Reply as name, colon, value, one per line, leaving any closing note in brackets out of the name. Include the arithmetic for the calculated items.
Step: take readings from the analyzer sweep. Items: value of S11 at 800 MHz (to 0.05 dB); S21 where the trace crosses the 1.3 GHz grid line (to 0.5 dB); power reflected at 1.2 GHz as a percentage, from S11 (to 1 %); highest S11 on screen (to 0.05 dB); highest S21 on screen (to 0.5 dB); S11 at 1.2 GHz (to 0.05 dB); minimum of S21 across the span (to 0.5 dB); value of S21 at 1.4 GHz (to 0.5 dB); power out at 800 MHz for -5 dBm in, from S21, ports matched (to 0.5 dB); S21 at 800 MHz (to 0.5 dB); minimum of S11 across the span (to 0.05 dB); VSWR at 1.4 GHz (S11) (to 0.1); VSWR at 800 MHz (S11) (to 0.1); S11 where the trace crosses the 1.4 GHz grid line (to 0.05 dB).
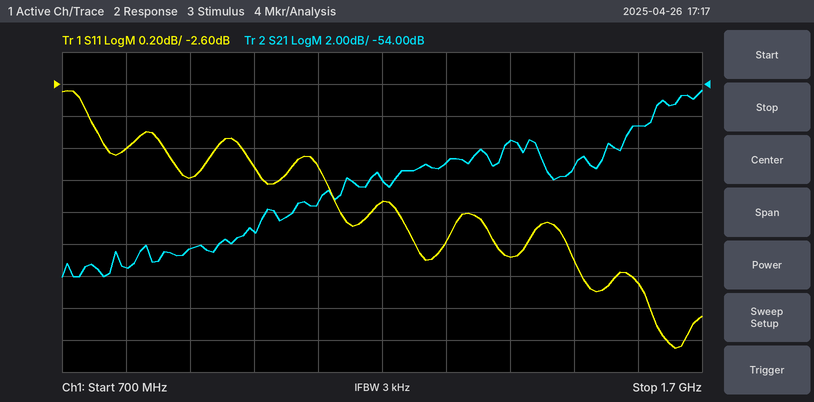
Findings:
value of S11 at 800 MHz: -3.00 dB
S21 where the trace crosses the 1.3 GHz grid line: -59.0 dB
power reflected at 1.2 GHz as a percentage, from S11: 10^(-3.35/10) ≈ 46 %
highest S11 on screen: -2.65 dB
highest S21 on screen: -54.5 dB
S11 at 1.2 GHz: -3.35 dB
minimum of S21 across the span: -66.0 dB
value of S21 at 1.4 GHz: -57.5 dB
power out at 800 MHz for -5 dBm in, from S21, ports matched: -5 dBm + (-65.5 dB) = -70.5 dBm
S21 at 800 MHz: -65.5 dB
minimum of S11 across the span: -4.25 dB
VSWR at 1.4 GHz (S11): |Γ| = 10^(-3.7/20) = 0.6531; VSWR = (1 + 0.6531)/(1 − 0.6531) ≈ 4.8
VSWR at 800 MHz (S11): |Γ| = 10^(-3/20) = 0.7079; VSWR = (1 + 0.7079)/(1 − 0.7079) ≈ 5.8
S11 where the trace crosses the 1.4 GHz grid line: -3.70 dB
